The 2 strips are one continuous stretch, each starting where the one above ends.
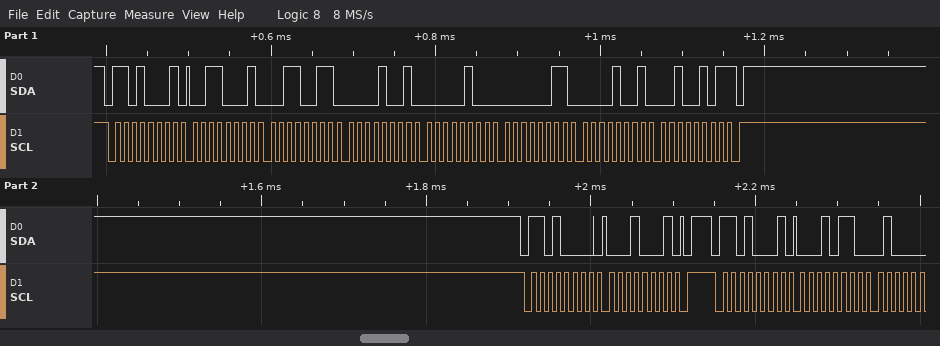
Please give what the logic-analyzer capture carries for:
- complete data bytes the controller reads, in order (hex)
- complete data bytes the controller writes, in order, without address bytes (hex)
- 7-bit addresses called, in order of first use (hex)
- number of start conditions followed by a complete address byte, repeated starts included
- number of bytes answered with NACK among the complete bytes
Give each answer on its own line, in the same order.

31 33 09 04 03 09 25 16
11
0x68
3
1
